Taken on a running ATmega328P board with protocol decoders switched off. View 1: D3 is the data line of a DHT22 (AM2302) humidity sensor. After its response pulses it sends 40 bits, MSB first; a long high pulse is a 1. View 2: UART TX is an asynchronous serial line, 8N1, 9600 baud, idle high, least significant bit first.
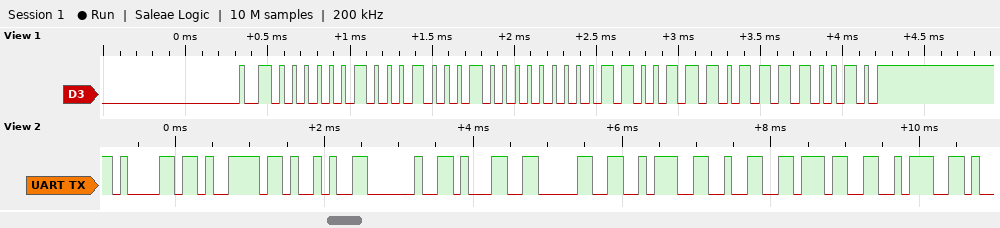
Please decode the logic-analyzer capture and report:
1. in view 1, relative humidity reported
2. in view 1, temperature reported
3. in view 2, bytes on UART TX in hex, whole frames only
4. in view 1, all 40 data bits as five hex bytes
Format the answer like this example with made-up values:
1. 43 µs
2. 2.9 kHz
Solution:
1. 54.6 %
2. 20.6 °C
3. 61 79 29 20 31 30 3A 32 37 3A
4. 02 22 00 CE F2
